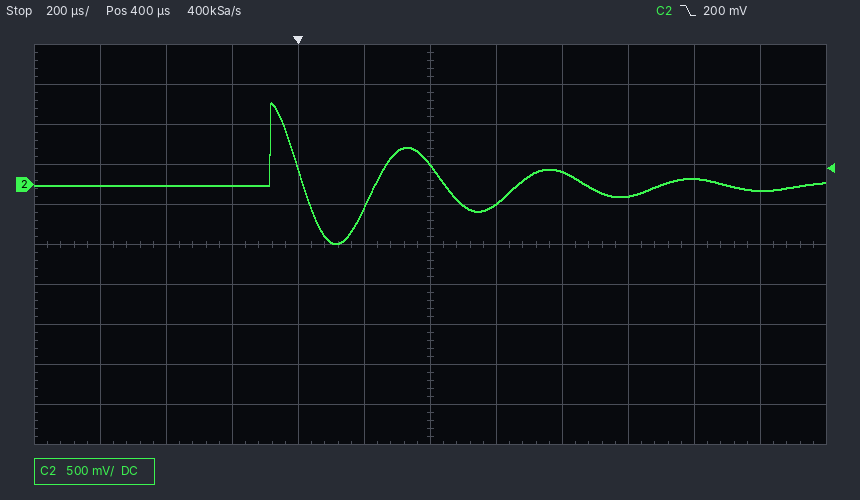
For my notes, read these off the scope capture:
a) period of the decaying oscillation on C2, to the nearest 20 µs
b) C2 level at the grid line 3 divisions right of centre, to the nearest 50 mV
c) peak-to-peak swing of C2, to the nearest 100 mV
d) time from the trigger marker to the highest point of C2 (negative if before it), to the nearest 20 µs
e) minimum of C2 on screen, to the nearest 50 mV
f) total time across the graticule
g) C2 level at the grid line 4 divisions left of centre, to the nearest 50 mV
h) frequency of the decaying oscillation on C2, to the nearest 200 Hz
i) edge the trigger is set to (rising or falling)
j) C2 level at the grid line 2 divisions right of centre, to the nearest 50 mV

420 µs
-150 mV
1.80 V
-80 µs
-750 mV
2.4 ms
0 mV
2.4 kHz
falling
150 mV
